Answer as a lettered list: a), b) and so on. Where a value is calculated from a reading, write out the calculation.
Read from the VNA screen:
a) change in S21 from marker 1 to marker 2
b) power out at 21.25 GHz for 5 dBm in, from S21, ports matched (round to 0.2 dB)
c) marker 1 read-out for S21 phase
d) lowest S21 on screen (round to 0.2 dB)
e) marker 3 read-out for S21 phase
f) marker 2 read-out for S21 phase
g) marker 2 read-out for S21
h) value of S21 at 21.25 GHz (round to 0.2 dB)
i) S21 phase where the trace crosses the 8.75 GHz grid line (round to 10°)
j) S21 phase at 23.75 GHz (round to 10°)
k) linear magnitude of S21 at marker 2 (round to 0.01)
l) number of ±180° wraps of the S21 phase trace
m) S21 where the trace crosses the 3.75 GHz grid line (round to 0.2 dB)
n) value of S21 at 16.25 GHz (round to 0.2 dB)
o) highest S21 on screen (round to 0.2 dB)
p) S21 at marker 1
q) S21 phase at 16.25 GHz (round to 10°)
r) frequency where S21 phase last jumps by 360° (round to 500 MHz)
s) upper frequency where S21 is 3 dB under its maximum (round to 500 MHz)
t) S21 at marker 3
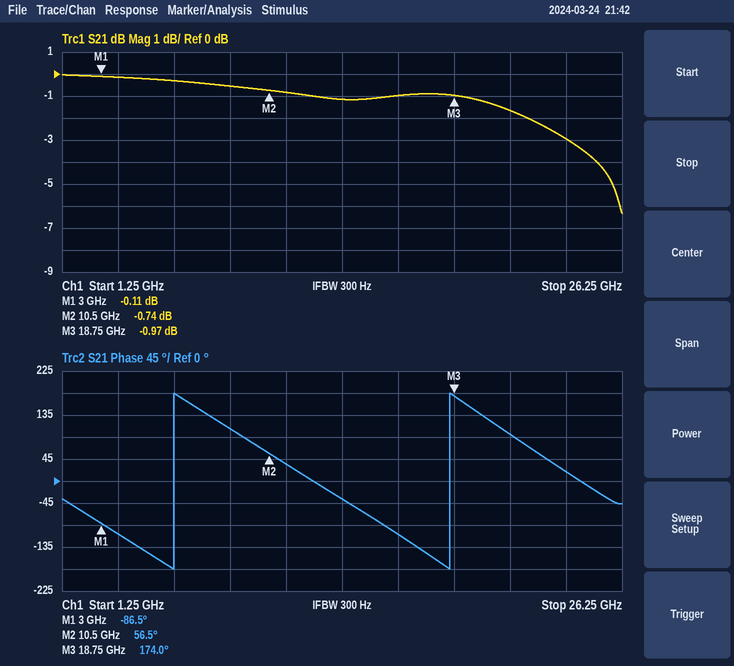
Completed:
a) -0.74 − (-0.11) = -0.63 dB
b) 5 dBm + (-1.6 dB) = 3.4 dBm
c) -86.5°
d) -6.4 dB
e) 174.0°
f) 56.5°
g) -0.74 dB
h) -1.6 dB
i) 110°
j) 20°
k) 10^(-0.74/20) ≈ 0.92
l) 2
m) -0.2 dB
n) -1.0 dB
o) 0.0 dB
p) -0.11 dB
q) -110°
r) 18.5 GHz
s) 24.0 GHz
t) -0.97 dB
